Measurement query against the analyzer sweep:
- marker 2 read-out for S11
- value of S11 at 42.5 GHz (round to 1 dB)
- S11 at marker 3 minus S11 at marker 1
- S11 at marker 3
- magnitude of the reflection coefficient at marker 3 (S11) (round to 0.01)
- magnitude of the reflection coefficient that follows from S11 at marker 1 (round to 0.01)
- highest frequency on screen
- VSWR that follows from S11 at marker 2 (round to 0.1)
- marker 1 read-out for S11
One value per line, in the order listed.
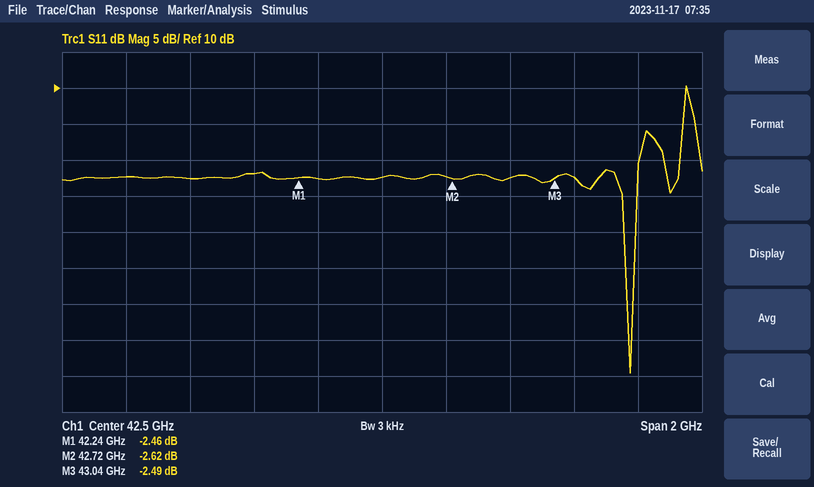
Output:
-2.62 dB
-2 dB
-0.03 dB
-2.49 dB
0.75
0.75
43.5 GHz
6.7
-2.46 dB
